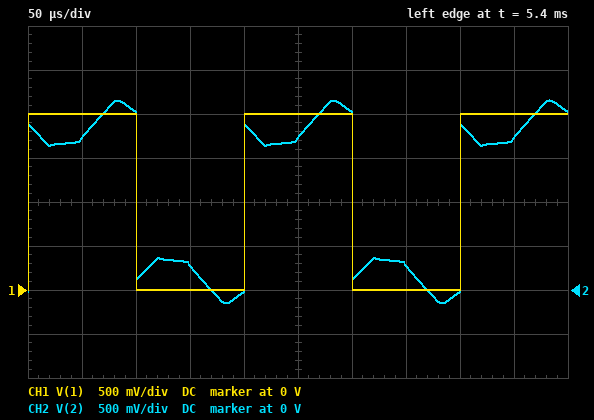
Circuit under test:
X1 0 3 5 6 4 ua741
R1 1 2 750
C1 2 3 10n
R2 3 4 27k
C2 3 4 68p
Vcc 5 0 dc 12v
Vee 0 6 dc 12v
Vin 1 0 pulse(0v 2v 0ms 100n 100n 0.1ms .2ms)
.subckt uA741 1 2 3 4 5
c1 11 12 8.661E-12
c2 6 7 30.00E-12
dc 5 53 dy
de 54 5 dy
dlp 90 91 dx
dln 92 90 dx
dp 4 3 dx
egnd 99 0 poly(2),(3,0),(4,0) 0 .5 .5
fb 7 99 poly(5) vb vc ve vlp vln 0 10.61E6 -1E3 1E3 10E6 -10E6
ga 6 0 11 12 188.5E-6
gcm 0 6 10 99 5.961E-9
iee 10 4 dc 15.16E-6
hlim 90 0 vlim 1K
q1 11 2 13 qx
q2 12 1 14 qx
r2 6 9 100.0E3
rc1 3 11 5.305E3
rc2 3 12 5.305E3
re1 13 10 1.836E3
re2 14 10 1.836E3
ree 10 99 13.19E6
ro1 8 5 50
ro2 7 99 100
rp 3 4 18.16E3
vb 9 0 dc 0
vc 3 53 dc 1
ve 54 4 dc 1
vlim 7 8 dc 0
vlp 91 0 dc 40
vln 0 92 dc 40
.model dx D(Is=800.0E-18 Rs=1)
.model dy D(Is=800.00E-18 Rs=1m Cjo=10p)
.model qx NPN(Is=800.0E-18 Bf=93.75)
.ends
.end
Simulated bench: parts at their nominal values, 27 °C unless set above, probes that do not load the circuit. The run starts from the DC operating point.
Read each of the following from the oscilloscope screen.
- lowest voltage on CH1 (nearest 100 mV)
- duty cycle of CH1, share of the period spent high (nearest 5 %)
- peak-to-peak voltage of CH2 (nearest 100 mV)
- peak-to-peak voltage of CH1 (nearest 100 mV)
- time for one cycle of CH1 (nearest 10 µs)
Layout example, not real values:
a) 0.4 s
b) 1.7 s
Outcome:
a) 0 V
b) 50 %
c) 2.3 V
d) 2.0 V
e) 200 µs
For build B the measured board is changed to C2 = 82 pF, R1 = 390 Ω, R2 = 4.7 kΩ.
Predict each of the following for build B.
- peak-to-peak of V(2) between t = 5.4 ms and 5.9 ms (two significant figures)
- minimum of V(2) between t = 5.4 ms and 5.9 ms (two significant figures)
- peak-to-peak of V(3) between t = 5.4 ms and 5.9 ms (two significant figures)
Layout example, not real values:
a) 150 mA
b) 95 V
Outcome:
a) 2.4 V
b) -190 mV
c) 3.6 V
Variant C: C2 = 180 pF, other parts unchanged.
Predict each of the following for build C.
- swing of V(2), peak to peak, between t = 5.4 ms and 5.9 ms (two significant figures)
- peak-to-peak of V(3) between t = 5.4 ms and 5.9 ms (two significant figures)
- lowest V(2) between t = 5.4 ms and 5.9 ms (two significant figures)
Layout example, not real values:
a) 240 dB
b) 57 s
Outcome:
a) 2.2 V
b) 3.6 V
c) -100 mV
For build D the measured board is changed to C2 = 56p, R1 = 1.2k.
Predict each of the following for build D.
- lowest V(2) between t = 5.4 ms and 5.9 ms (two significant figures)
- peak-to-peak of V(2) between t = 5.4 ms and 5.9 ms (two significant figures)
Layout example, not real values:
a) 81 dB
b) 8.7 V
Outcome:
a) -110 mV
b) 2.2 V
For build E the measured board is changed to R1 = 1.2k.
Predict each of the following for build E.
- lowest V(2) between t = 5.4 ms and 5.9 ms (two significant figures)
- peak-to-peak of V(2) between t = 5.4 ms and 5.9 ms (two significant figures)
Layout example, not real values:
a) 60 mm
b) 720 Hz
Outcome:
a) -97 mV
b) 2.2 V
